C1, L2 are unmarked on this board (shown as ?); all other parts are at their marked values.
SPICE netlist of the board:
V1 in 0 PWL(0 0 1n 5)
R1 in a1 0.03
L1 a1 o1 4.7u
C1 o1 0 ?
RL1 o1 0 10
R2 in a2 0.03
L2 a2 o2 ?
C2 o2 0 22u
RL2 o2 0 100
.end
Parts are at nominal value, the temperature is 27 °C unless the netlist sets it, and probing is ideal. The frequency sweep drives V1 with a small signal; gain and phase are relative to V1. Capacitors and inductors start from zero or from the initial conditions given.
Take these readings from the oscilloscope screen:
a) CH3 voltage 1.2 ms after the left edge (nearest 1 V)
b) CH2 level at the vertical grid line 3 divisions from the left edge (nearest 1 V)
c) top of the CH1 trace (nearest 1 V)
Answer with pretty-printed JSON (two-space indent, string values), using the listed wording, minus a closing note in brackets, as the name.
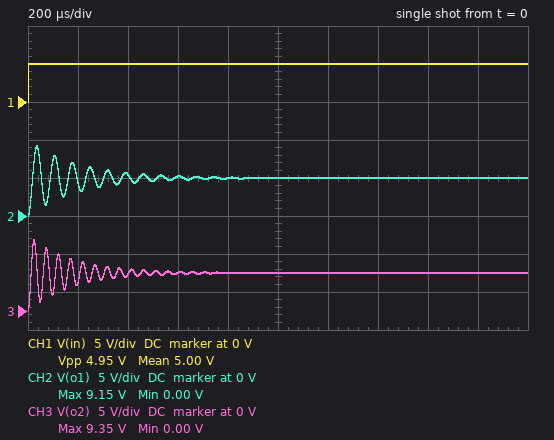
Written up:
{
  "CH3 voltage 1.2 ms after the left edge": "5 V",
  "CH2 level at the vertical grid line 3 divisions from the left edge": "5 V",
  "top of the CH1 trace": "5 V"
}
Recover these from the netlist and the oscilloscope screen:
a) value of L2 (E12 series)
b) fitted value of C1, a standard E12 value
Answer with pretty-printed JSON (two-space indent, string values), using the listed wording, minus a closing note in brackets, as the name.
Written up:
{
  "value of L2": "2.7 µH",
  "fitted value of C1, a standard E12 value": "27 µF"
}
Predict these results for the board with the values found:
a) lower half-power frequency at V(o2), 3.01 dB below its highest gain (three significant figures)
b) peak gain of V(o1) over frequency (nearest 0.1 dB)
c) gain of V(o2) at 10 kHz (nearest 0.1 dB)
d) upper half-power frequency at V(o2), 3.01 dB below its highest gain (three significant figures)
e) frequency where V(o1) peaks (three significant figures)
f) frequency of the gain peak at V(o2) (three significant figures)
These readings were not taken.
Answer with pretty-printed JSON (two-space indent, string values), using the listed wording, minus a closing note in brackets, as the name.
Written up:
{
  "lower half-power frequency at V(o2), 3.01 dB below its highest gain": "19.7 kHz",
  "peak gain of V(o1) over frequency": "18.9 dB",
  "gain of V(o2) at 10 kHz": "2.3 dB",
  "upper half-power frequency at V(o2), 3.01 dB below its highest gain": "21.5 kHz",
  "frequency where V(o1) peaks": "14.1 kHz",
  "frequency of the gain peak at V(o2)": "20.6 kHz"
}
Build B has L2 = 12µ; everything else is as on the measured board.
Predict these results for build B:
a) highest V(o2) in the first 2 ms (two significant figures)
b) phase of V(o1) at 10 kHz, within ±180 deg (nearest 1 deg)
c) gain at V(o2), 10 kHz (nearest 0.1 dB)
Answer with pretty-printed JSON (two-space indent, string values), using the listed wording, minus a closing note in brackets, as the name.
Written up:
{
  "highest V(o2) in the first 2 ms": "9.6 V",
  "phase of V(o1) at 10 kHz, within ±180 deg": "-9 deg",
  "gain at V(o2), 10 kHz": "23.8 dB"
}
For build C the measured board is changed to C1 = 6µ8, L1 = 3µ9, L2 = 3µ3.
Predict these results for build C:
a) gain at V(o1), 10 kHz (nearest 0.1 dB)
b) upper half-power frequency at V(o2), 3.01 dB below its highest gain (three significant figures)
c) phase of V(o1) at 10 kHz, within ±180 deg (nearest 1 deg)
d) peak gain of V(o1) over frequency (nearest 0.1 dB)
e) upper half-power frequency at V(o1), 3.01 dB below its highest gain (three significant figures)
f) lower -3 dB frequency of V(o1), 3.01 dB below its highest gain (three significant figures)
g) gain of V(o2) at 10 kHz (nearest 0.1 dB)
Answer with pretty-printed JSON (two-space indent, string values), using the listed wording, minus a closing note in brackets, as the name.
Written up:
{
  "gain at V(o1), 10 kHz": "0.9 dB",
  "upper half-power frequency at V(o2), 3.01 dB below its highest gain": "19.4 kHz",
  "phase of V(o1) at 10 kHz, within ±180 deg": "-2 deg",
  "peak gain of V(o1) over frequency": "18.8 dB",
  "upper half-power frequency at V(o1), 3.01 dB below its highest gain": "32.6 kHz",
  "lower -3 dB frequency of V(o1), 3.01 dB below its highest gain": "29.0 kHz",
  "gain of V(o2) at 10 kHz": "2.9 dB"
}
